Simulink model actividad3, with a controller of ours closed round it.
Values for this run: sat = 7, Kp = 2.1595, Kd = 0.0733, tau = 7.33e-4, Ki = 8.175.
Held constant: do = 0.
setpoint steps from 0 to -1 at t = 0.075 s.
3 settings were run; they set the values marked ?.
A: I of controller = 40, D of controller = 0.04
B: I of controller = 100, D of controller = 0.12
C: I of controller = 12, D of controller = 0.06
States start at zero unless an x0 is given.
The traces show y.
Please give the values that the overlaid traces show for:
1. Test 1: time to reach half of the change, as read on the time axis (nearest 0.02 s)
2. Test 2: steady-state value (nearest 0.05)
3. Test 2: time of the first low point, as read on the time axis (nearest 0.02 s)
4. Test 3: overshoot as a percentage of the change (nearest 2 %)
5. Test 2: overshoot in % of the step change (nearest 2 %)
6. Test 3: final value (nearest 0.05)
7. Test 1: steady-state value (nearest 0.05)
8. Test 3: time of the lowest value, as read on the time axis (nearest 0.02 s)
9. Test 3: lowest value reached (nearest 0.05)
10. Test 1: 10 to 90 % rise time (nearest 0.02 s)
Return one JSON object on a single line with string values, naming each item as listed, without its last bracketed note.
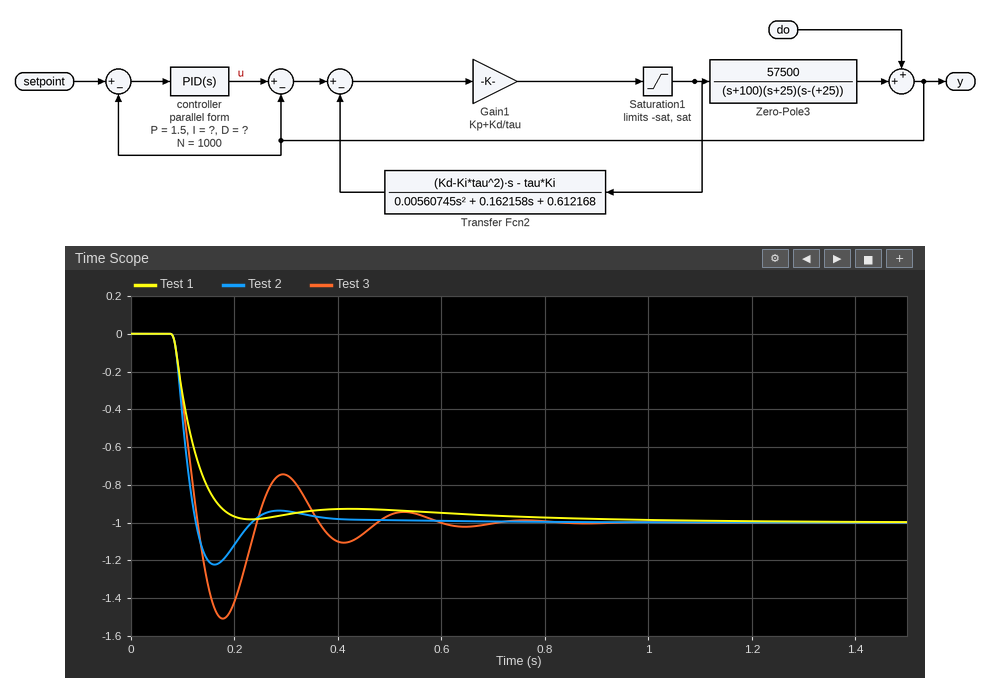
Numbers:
{"Test 1: time to reach half of the change, as read on the time axis": "0.12 s", "Test 2: steady-state value": "-1.00", "Test 2: time of the first low point, as read on the time axis": "0.16 s", "Test 3: overshoot as a percentage of the change": "50 %", "Test 2: overshoot in % of the step change": "22 %", "Test 3: final value": "-1.00", "Test 1: steady-state value": "-1.00", "Test 3: time of the lowest value, as read on the time axis": "0.18 s", "Test 3: lowest value reached": "-1.50", "Test 1: 10 to 90 % rise time": "0.08 s"}
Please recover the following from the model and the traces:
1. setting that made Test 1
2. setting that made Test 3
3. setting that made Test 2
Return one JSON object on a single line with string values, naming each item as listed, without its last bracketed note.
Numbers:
{"setting that made Test 1": "C", "setting that made Test 3": "B", "setting that made Test 2": "A"}
